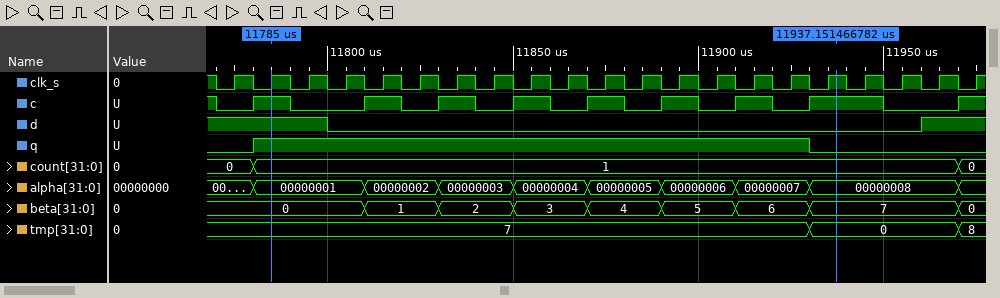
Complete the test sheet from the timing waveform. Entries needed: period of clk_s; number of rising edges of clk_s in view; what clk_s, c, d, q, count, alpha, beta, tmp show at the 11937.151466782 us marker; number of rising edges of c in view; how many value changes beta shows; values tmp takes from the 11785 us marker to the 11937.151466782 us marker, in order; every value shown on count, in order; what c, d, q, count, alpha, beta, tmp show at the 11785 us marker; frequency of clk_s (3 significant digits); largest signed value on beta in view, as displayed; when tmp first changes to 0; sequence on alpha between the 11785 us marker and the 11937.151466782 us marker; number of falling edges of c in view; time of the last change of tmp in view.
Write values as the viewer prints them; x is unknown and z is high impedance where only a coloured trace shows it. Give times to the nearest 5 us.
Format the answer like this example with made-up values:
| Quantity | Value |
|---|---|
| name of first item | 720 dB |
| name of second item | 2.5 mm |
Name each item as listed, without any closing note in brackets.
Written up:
| Quantity | Value |
|---|---|
| period of clk_s | 10 us |
| number of rising edges of clk_s in view | 21 |
| what clk_s, c, d, q, count, alpha, beta, tmp show at the 11937.151466782 us marker | clk_s=1, c=1, d=0, q=0, count=1, alpha=00000008, beta=7, tmp=0 |
| number of rising edges of c in view | 9 |
| how many value changes beta shows | 8 |
| values tmp takes from the 11785 us marker to the 11937.151466782 us marker, in order | 7, 0 |
| every value shown on count, in order | 0, 1, 0 |
| what c, d, q, count, alpha, beta, tmp show at the 11785 us marker | c=1, d=1, q=1, count=1, alpha=00000001, beta=0, tmp=7 |
| frequency of clk_s | 100 kHz |
| largest signed value on beta in view, as displayed | 7 |
| when tmp first changes to 0 | 11930 us |
| sequence on alpha between the 11785 us marker and the 11937.151466782 us marker | 00000001, 00000002, 00000003, 00000004, 00000005, 00000006, 00000007, 00000008 |
| number of falling edges of c in view | 9 |
| time of the last change of tmp in view | 11970 us |
